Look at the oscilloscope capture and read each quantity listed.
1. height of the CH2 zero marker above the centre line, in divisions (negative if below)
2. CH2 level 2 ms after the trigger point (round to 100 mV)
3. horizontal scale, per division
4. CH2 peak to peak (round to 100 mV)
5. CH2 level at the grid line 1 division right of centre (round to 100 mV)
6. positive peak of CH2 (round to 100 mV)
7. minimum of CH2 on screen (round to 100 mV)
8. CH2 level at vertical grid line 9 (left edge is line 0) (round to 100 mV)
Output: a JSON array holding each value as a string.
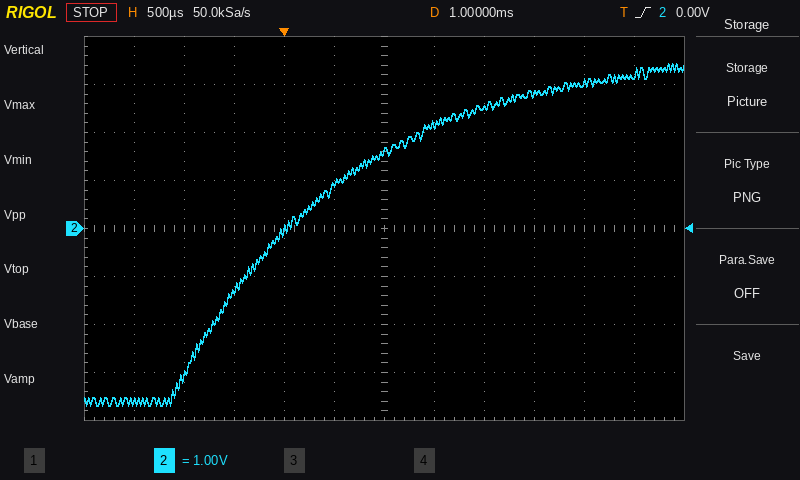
["0.0 div", "2.5 V", "500 µs", "7.1 V", "2.2 V", "3.4 V", "-3.7 V", "2.8 V"]
